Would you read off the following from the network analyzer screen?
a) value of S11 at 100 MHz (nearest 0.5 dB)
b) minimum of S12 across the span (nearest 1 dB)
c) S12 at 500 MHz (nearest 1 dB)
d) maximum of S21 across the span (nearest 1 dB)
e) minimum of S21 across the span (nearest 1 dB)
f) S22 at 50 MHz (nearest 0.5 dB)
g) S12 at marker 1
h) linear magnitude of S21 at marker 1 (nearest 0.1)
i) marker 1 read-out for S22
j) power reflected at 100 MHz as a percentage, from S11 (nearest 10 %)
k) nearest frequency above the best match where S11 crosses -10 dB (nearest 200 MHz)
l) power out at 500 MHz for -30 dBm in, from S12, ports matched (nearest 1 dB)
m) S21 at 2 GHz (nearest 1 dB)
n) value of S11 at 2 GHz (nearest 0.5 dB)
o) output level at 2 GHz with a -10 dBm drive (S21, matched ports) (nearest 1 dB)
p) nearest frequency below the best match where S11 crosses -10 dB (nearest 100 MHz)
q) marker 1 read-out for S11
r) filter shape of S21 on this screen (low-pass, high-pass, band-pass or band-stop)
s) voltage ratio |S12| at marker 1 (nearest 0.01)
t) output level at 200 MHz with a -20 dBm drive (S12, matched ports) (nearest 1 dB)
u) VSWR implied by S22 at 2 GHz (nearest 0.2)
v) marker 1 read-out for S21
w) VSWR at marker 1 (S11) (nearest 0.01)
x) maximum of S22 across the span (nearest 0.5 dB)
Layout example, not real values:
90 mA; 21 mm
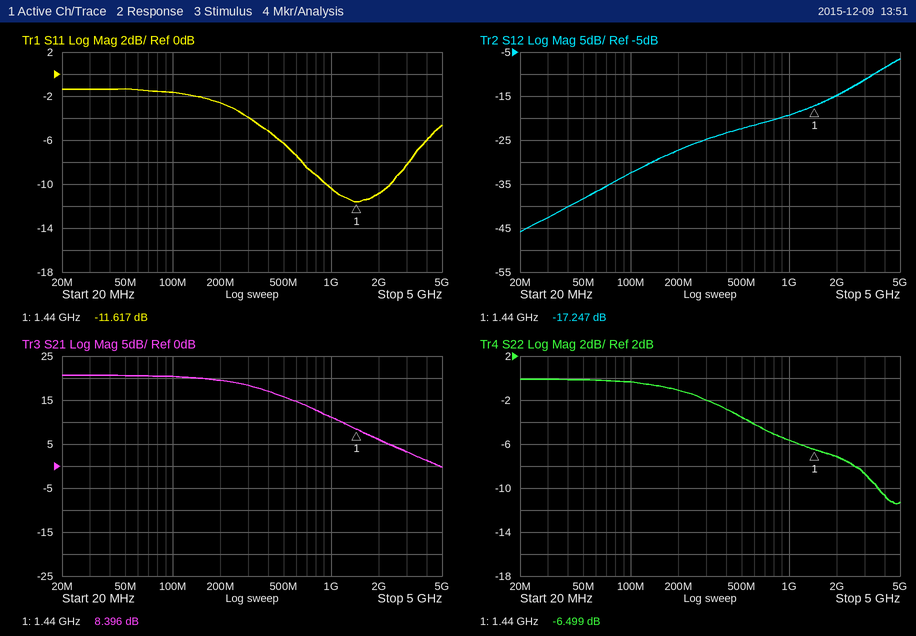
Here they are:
-1.5 dB; -46 dB; -22 dB; 21 dB; 0 dB; 0.0 dB; -17.247 dB; 2.6; -6.499 dB; 70 %; 2.4 GHz; -52 dBm; 6 dB; -11.0 dB; -4 dBm; 900 MHz; -11.617 dB; low-pass; 0.14; -47 dBm; 2.6; 8.396 dB; 1.71; 0.0 dB
